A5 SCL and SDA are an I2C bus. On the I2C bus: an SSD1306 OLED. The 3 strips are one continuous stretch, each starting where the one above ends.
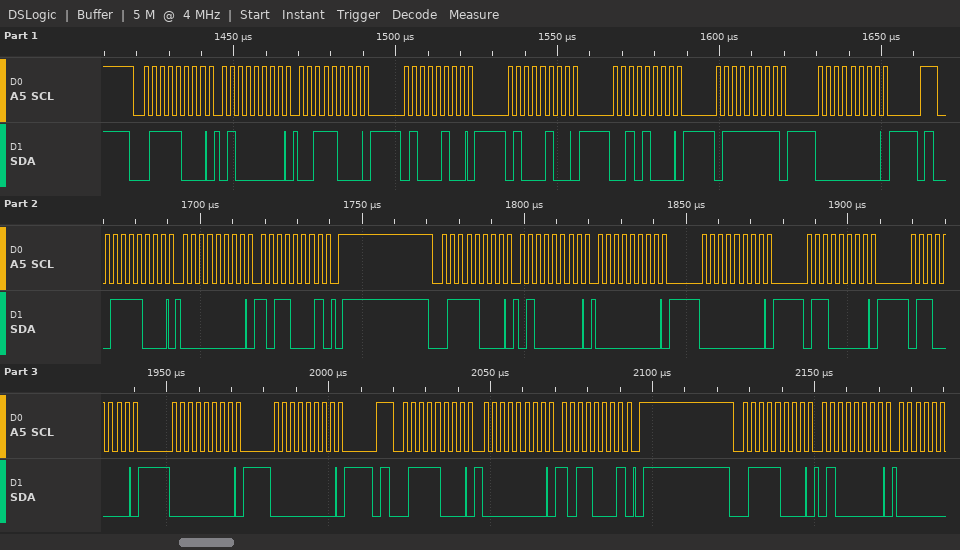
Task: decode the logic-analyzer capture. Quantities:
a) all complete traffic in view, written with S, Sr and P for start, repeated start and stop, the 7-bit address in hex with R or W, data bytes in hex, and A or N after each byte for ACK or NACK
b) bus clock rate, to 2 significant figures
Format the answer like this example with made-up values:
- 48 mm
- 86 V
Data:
- S 3CW A 40 A 38 A 44 A 44 A 28 A 7F A 00 A P S 3CW A 00 A B1 A P S 3CW A 40 A 00 A 00 A 60 A 60 A 00 A 00 A P S 3CW A 00 A B1 A P S 3CW A 40 A
- 400 kHz
